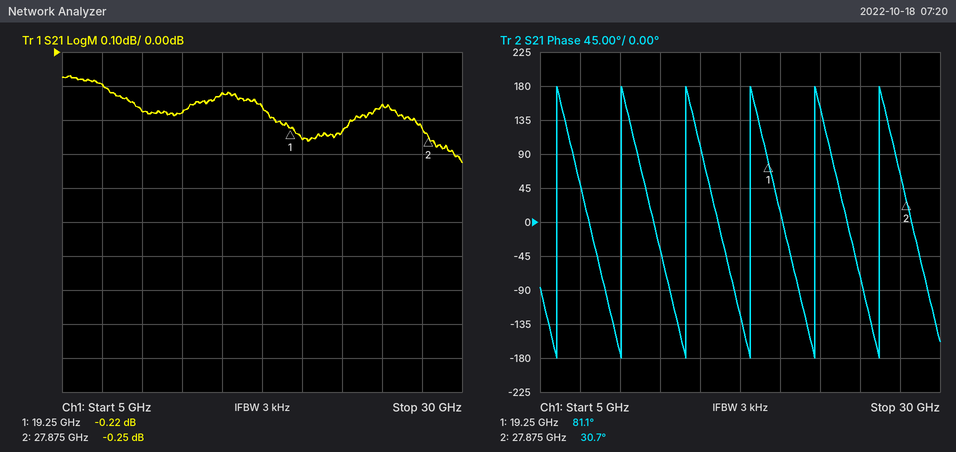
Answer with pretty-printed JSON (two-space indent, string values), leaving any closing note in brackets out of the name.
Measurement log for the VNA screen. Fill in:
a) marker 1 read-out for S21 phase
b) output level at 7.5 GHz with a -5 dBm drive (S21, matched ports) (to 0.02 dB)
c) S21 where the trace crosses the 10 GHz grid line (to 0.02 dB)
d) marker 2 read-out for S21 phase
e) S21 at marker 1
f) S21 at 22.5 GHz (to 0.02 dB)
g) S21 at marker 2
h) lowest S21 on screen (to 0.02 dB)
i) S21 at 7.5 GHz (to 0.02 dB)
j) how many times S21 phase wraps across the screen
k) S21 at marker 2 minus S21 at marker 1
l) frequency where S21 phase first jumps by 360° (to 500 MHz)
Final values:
{
  "marker 1 read-out for S21 phase": "81.1°",
  "output level at 7.5 GHz with a -5 dBm drive (S21, matched ports)": "-5.10 dBm",
  "S21 where the trace crosses the 10 GHz grid line": "-0.18 dB",
  "marker 2 read-out for S21 phase": "30.7°",
  "S21 at marker 1": "-0.22 dB",
  "S21 at 22.5 GHz": "-0.24 dB",
  "S21 at marker 2": "-0.25 dB",
  "lowest S21 on screen": "-0.32 dB",
  "S21 at 7.5 GHz": "-0.10 dB",
  "how many times S21 phase wraps across the screen": "6",
  "S21 at marker 2 minus S21 at marker 1": "-0.03 dB",
  "frequency where S21 phase first jumps by 360°": "6.0 GHz"
}
